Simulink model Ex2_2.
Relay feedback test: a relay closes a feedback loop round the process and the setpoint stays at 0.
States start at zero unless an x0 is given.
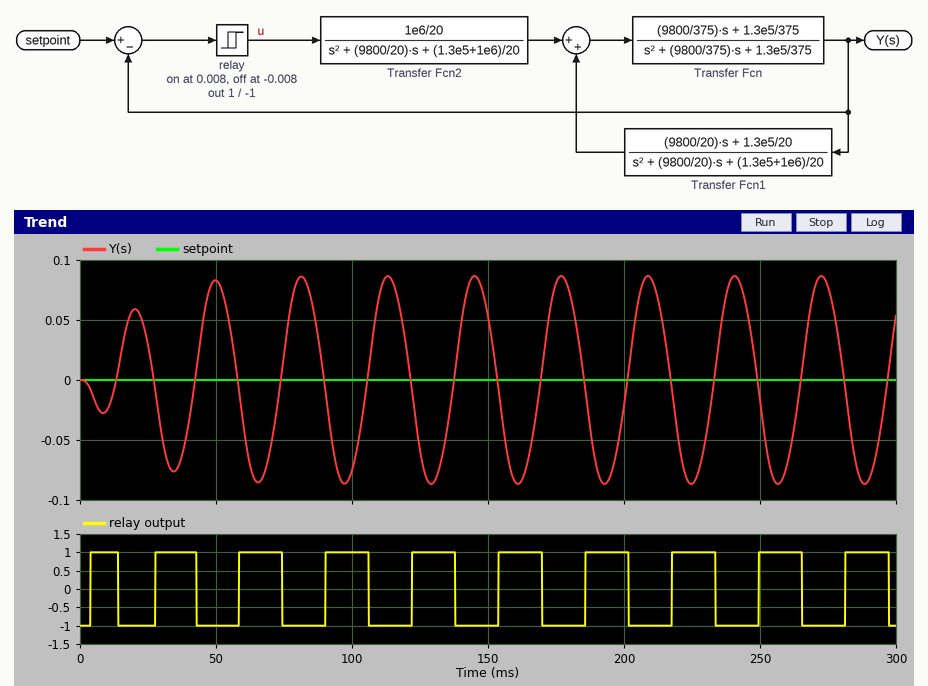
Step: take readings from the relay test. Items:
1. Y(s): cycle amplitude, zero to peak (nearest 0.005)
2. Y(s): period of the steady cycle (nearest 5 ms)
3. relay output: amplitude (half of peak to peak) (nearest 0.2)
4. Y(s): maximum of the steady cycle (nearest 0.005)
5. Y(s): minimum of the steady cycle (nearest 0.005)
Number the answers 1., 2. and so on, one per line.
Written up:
1. 0.085
2. 30 ms
3. 1.0
4. 0.085
5. -0.085
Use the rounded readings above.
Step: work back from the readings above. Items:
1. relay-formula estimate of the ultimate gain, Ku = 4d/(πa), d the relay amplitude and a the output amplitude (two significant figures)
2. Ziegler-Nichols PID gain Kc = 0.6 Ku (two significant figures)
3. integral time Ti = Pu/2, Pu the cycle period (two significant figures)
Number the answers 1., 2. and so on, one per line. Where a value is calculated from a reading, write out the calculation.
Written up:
1. 4 × 1 / (π × 0.085) = 15
2. 0.6 × 15 = 9.0
3. 30 / 2 = 15 ms
